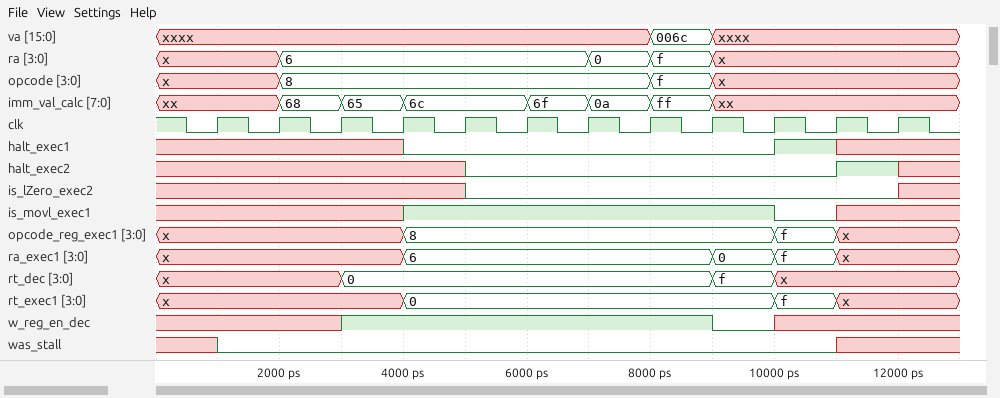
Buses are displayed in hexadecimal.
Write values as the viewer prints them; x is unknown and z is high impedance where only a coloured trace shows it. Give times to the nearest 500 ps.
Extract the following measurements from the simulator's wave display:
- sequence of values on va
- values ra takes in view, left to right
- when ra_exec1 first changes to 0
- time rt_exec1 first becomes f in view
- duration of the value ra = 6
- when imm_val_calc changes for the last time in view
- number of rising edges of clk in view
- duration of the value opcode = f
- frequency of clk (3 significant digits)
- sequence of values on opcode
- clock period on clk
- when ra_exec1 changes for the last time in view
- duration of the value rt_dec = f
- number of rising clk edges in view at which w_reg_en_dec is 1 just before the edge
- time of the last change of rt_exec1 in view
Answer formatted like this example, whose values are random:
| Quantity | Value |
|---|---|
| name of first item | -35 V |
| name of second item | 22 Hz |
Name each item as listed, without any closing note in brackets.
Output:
| Quantity | Value |
|---|---|
| sequence of values on va | xxxx, 006c, xxxx |
| values ra takes in view, left to right | x, 6, 0, f, x |
| when ra_exec1 first changes to 0 | 9000 ps |
| time rt_exec1 first becomes f in view | 10000 ps |
| duration of the value ra = 6 | 5000 ps |
| when imm_val_calc changes for the last time in view | 9000 ps |
| number of rising edges of clk in view | 12 |
| duration of the value opcode = f | 1000 ps |
| frequency of clk | 1.00 GHz |
| sequence of values on opcode | x, 8, f, x |
| clock period on clk | 1000 ps |
| when ra_exec1 changes for the last time in view | 11000 ps |
| duration of the value rt_dec = f | 1000 ps |
| number of rising clk edges in view at which w_reg_en_dec is 1 just before the edge | 6 |
| time of the last change of rt_exec1 in view | 11000 ps |
